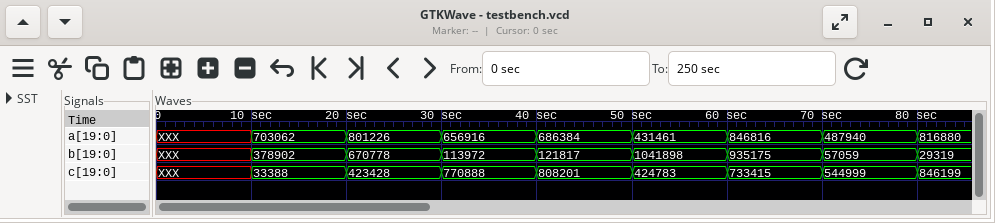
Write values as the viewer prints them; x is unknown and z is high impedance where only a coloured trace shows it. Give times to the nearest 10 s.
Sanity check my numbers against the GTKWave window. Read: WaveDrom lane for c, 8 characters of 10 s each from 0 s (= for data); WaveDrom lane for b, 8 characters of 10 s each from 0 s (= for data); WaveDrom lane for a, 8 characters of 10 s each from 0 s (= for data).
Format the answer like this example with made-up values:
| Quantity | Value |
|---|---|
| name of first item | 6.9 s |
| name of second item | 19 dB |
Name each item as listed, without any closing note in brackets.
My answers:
| Quantity | Value |
|---|---|
| WaveDrom lane for c, 8 characters of 10 s each from 0 s | {name: 'c', wave: 'x=======', data: '33388 423428 770888 808201 424783 733415 544999'} |
| WaveDrom lane for b, 8 characters of 10 s each from 0 s | {name: 'b', wave: 'x=======', data: '378902 670778 113972 121817 1041898 935175 57059'} |
| WaveDrom lane for a, 8 characters of 10 s each from 0 s | {name: 'a', wave: 'x=======', data: '703062 801226 656916 686384 431461 846816 487940'} |
